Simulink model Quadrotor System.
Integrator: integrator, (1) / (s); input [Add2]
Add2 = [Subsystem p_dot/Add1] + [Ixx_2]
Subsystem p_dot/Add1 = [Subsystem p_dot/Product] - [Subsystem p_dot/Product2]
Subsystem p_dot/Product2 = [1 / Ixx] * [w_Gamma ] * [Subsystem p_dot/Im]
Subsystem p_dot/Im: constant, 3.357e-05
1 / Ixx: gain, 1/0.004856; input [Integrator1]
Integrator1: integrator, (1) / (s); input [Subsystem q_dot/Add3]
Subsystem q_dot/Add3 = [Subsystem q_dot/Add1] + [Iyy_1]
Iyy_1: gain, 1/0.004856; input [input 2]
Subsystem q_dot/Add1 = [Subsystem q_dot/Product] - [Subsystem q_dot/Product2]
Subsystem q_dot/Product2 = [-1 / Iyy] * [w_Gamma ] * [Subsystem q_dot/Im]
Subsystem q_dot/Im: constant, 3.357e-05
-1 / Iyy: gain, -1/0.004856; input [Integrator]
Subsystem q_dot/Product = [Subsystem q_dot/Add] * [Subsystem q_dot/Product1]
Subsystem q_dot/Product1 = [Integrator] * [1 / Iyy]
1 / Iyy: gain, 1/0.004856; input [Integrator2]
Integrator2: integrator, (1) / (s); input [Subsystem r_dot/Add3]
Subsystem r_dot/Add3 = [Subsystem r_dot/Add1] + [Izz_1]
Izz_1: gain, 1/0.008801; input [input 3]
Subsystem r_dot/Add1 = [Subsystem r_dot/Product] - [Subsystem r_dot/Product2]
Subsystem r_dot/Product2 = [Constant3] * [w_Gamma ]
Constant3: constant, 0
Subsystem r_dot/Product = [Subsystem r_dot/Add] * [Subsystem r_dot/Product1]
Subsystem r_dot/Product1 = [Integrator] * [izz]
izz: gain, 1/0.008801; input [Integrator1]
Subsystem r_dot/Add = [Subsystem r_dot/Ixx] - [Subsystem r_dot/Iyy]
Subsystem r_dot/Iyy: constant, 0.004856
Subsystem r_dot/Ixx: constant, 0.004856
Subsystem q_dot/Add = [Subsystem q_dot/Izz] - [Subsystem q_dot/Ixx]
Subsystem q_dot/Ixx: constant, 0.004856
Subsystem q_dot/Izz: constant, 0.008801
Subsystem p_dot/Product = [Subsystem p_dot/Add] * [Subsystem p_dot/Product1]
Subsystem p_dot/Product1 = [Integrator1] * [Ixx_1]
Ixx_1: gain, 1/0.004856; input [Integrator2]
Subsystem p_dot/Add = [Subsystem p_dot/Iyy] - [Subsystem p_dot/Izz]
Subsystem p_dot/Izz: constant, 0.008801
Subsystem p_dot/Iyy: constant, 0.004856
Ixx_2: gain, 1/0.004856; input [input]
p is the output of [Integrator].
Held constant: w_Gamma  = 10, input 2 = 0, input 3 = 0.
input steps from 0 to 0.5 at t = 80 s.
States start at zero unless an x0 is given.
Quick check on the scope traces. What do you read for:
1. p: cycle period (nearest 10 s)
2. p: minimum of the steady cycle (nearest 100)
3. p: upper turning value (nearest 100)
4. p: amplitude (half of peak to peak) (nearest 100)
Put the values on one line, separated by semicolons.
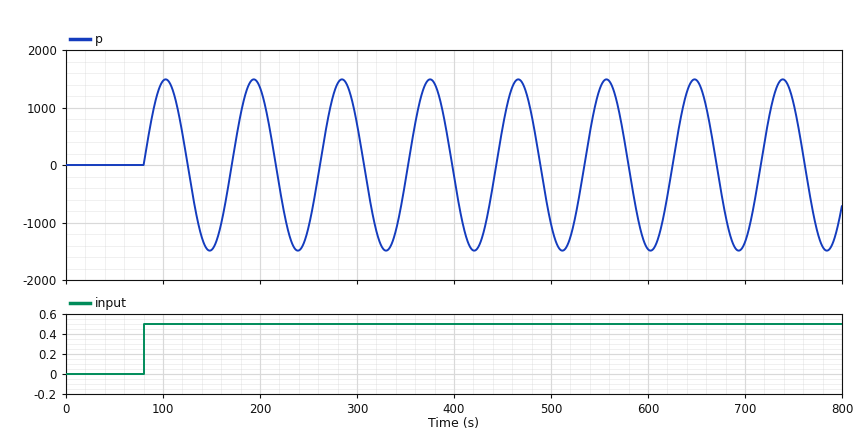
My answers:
90 s; -1500; 1500; 1500
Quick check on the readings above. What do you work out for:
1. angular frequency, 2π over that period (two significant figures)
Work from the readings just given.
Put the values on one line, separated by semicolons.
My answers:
0.070 rad/s
